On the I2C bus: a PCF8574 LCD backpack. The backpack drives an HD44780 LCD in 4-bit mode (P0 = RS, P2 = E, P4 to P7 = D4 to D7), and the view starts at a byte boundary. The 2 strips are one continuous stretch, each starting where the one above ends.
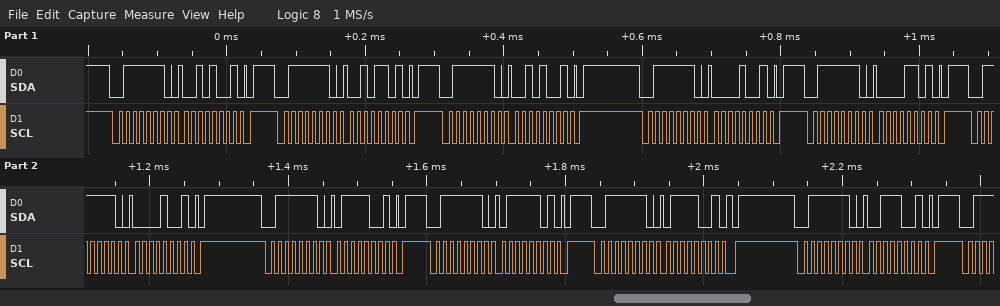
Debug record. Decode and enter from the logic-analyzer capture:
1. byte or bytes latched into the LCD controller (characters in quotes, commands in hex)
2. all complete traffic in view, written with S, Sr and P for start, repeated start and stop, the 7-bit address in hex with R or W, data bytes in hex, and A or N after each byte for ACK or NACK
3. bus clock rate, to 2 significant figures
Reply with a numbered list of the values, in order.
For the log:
1. ' '
2. S 3FW A 29 A P S 3FW A 2D A P S 3FW A 29 A P S 3FW A 09 A P S 3FW A 0D A P S 3FW A 09 A P S 3FW A 79 A P S 3FW A 7D A P S 3FW A 79 A P S 3FW A 39 A P
3. 100 kHz
